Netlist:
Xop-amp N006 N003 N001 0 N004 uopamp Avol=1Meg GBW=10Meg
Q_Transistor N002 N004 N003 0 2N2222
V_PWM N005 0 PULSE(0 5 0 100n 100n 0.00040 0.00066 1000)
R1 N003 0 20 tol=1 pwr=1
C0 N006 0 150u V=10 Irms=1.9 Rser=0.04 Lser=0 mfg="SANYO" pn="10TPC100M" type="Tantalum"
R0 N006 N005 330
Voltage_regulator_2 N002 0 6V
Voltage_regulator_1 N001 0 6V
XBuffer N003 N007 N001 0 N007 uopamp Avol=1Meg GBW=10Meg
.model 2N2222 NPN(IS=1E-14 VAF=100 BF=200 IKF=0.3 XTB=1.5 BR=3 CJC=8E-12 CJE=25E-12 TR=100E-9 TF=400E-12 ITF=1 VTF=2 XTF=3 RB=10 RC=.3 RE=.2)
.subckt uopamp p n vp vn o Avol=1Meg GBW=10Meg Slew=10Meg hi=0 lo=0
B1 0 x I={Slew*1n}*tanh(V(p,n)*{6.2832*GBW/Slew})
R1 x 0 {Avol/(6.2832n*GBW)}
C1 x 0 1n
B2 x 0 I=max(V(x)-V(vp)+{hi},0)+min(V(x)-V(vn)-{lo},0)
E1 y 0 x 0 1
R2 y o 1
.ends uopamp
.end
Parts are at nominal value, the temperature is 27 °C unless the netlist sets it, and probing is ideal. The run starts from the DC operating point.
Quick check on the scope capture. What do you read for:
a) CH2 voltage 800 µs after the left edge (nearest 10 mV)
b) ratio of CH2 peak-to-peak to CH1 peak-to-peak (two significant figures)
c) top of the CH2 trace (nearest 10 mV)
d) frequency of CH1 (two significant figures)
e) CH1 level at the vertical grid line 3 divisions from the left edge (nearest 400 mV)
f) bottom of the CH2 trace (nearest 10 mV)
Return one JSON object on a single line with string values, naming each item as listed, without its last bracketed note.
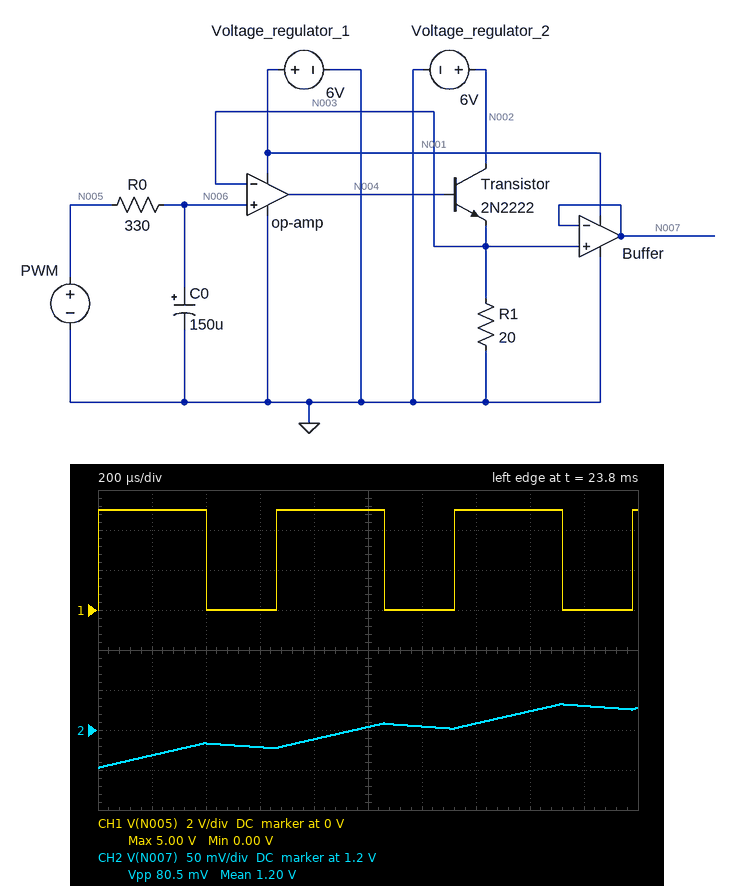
{"CH2 voltage 800 µs after the left edge": "1.19 V", "ratio of CH2 peak-to-peak to CH1 peak-to-peak": "0.016", "top of the CH2 trace": "1.23 V", "frequency of CH1": "1.5 kHz", "CH1 level at the vertical grid line 3 divisions from the left edge": "0 V", "bottom of the CH2 trace": "1.15 V"}
